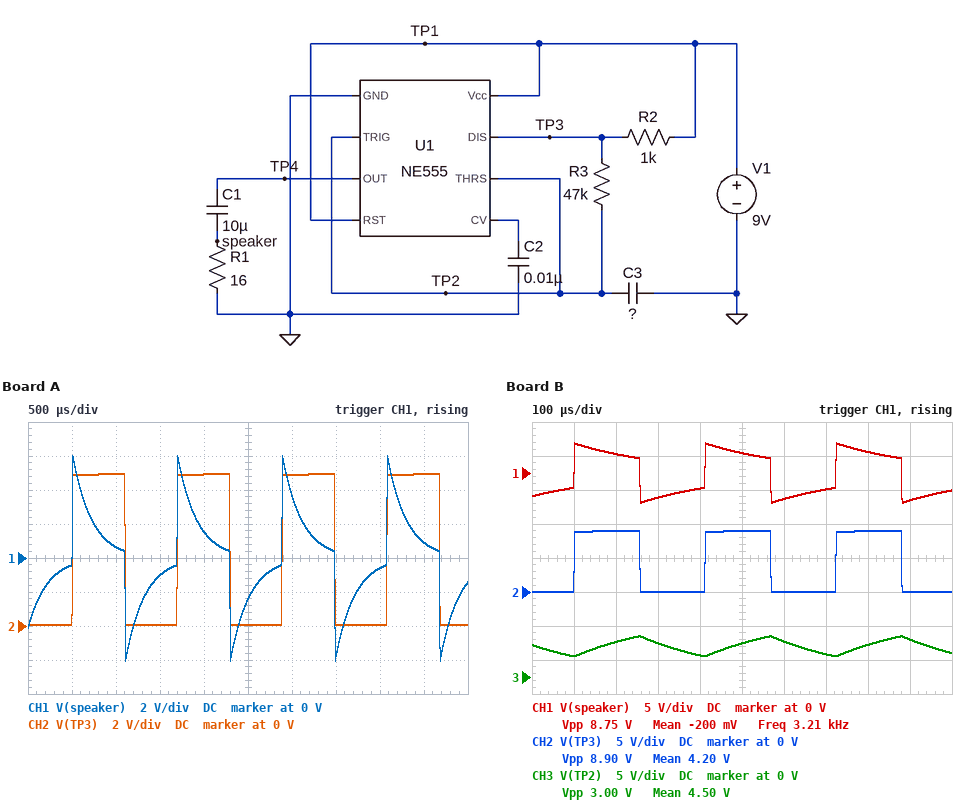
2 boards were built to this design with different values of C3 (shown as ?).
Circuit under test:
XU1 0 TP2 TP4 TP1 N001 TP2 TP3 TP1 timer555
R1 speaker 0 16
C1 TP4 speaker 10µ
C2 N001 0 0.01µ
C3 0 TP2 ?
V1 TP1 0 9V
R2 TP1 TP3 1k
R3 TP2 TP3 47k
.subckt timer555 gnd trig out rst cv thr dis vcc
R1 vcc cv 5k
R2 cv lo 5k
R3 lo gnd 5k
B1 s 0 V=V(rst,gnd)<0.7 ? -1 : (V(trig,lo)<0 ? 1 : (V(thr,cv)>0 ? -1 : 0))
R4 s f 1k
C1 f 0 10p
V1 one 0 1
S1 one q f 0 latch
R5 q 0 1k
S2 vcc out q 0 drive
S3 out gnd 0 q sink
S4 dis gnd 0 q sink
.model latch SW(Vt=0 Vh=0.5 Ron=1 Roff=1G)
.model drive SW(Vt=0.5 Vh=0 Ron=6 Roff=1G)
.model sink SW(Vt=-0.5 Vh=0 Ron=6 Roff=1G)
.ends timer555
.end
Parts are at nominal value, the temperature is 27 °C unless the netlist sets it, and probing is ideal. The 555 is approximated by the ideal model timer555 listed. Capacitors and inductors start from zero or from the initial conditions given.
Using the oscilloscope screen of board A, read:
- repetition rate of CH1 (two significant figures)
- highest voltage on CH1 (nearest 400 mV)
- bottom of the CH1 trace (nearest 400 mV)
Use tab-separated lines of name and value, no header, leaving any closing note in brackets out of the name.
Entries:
repetition rate of CH1	840 Hz
highest voltage on CH1	6.0 V
bottom of the CH1 trace	-6.0 V
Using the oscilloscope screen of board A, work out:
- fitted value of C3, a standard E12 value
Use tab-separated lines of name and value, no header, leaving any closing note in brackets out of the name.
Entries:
fitted value of C3, a standard E12 value	18 nF
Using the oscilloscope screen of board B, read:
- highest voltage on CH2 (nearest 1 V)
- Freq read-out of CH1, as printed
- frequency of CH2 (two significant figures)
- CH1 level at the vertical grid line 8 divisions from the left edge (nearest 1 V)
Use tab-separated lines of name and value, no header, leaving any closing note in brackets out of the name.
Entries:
highest voltage on CH2	9 V
Freq read-out of CH1, as printed	3.21 kHz
frequency of CH2	3.2 kHz
CH1 level at the vertical grid line 8 divisions from the left edge	3 V
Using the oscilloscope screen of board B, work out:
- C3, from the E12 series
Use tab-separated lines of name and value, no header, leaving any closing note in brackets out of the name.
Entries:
C3, from the E12 series	4.7 nF
